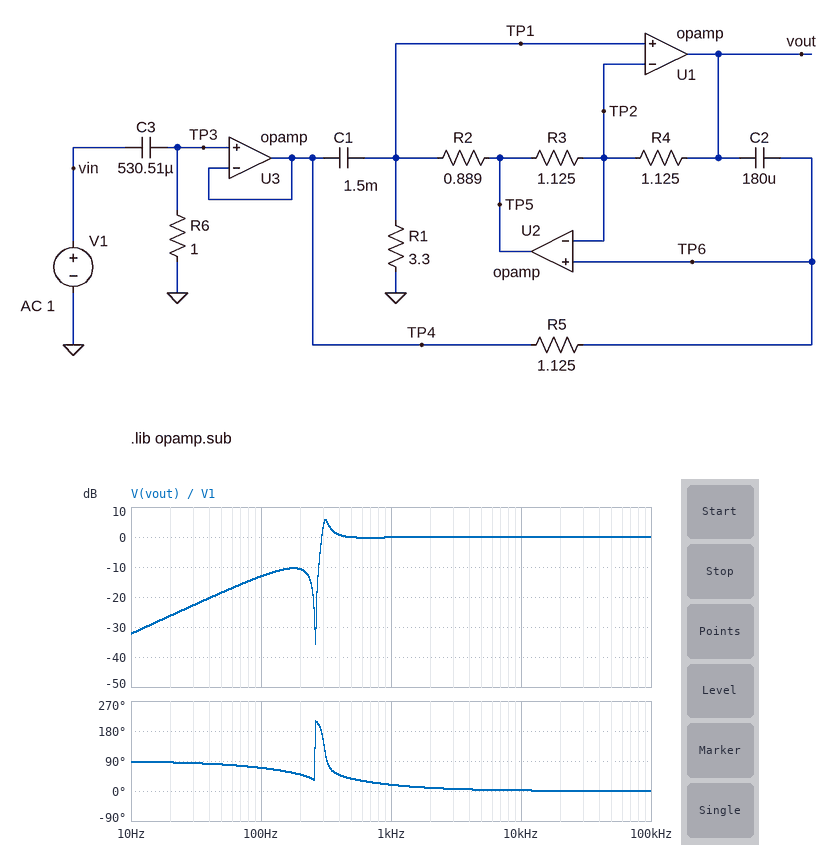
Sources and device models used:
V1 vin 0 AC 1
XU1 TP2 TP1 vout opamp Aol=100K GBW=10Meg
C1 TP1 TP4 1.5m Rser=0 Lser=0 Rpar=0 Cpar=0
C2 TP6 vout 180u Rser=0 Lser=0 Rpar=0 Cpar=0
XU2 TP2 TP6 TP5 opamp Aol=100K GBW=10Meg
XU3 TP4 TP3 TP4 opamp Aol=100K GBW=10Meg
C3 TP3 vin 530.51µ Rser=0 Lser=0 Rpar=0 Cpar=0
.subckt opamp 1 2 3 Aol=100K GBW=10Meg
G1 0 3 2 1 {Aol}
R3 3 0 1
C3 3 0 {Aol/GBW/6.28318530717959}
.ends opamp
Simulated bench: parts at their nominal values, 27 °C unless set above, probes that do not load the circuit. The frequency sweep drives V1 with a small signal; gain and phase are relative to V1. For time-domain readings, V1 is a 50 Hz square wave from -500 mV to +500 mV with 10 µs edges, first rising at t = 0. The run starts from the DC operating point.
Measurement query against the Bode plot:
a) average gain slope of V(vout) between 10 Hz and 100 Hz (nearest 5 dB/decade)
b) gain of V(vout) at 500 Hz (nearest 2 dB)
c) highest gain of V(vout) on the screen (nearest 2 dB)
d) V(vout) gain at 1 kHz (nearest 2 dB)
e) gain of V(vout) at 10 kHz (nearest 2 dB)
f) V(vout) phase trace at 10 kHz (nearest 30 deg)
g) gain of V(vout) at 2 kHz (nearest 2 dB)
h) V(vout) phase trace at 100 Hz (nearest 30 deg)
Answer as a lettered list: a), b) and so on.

a) 20 dB/decade
b) 0 dB
c) 6 dB
d) 0 dB
e) 0 dB
f) 0 deg
g) 0 dB
h) 60 deg
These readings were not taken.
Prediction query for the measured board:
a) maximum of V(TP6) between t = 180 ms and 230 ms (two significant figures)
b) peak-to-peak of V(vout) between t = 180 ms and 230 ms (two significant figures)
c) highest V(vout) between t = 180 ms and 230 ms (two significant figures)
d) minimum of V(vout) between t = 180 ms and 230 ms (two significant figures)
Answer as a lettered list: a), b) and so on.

a) 1.0 V
b) 2.0 V
c) 980 mV
d) -980 mV
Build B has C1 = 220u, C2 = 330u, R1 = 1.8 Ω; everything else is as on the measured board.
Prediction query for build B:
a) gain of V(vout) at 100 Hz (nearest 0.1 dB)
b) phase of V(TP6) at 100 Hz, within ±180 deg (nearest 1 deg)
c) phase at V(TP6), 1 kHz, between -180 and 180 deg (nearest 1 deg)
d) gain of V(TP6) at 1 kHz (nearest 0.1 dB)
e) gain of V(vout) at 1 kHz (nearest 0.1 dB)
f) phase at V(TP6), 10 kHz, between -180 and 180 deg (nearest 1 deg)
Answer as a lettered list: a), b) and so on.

a) -16.2 dB
b) 65 deg
c) 48 deg
d) -1.8 dB
e) 0.3 dB
f) 4 deg
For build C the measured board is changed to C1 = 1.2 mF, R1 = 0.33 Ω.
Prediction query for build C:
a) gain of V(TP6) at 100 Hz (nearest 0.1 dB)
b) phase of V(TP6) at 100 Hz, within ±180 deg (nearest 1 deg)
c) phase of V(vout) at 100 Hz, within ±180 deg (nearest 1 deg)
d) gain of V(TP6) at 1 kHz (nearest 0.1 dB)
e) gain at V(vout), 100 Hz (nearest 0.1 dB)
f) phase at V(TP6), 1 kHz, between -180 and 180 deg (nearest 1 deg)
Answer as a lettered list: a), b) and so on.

a) -10.6 dB
b) 51 deg
c) -129 deg
d) -1.2 dB
e) -4.8 dB
f) 41 deg
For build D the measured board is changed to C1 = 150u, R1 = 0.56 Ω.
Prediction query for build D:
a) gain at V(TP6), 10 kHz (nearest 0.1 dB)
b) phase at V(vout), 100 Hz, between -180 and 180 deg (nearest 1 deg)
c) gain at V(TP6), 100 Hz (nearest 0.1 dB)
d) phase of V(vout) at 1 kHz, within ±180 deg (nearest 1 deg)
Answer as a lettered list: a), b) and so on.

a) -0.2 dB
b) -120 deg
c) -10.2 dB
d) 105 deg
